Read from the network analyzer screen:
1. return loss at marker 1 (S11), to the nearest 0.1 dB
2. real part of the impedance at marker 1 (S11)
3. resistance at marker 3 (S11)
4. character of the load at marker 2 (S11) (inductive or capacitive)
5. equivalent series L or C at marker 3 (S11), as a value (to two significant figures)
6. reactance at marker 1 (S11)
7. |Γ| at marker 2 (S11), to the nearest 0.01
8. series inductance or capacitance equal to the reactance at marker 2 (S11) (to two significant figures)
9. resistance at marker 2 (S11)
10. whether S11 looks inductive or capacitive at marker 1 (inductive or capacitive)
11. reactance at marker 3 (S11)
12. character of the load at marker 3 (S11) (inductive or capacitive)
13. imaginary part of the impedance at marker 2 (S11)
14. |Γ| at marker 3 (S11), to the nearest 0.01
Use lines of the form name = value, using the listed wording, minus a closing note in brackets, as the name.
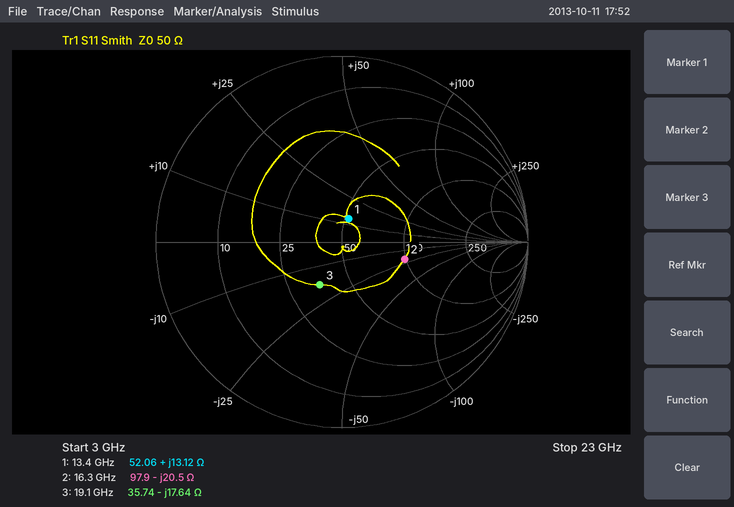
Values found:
return loss at marker 1 (S11), to the nearest 0.1 dB = 17.8 dB
real part of the impedance at marker 1 = 52.06 Ω
resistance at marker 3 = 35.74 Ω
character of the load at marker 2 (S11) = capacitive
equivalent series L or C at marker 3 (S11), as a value = 470 fF
reactance at marker 1 = +13.12 Ω
|Γ| at marker 2 (S11), to the nearest 0.01 = 0.35
series inductance or capacitance equal to the reactance at marker 2 (S11) = 480 fF
resistance at marker 2 = 97.9 Ω
whether S11 looks inductive or capacitive at marker 1 = inductive
reactance at marker 3 = -17.64 Ω
character of the load at marker 3 (S11) = capacitive
imaginary part of the impedance at marker 2 = -20.5 Ω
|Γ| at marker 3 (S11), to the nearest 0.01 = 0.26
